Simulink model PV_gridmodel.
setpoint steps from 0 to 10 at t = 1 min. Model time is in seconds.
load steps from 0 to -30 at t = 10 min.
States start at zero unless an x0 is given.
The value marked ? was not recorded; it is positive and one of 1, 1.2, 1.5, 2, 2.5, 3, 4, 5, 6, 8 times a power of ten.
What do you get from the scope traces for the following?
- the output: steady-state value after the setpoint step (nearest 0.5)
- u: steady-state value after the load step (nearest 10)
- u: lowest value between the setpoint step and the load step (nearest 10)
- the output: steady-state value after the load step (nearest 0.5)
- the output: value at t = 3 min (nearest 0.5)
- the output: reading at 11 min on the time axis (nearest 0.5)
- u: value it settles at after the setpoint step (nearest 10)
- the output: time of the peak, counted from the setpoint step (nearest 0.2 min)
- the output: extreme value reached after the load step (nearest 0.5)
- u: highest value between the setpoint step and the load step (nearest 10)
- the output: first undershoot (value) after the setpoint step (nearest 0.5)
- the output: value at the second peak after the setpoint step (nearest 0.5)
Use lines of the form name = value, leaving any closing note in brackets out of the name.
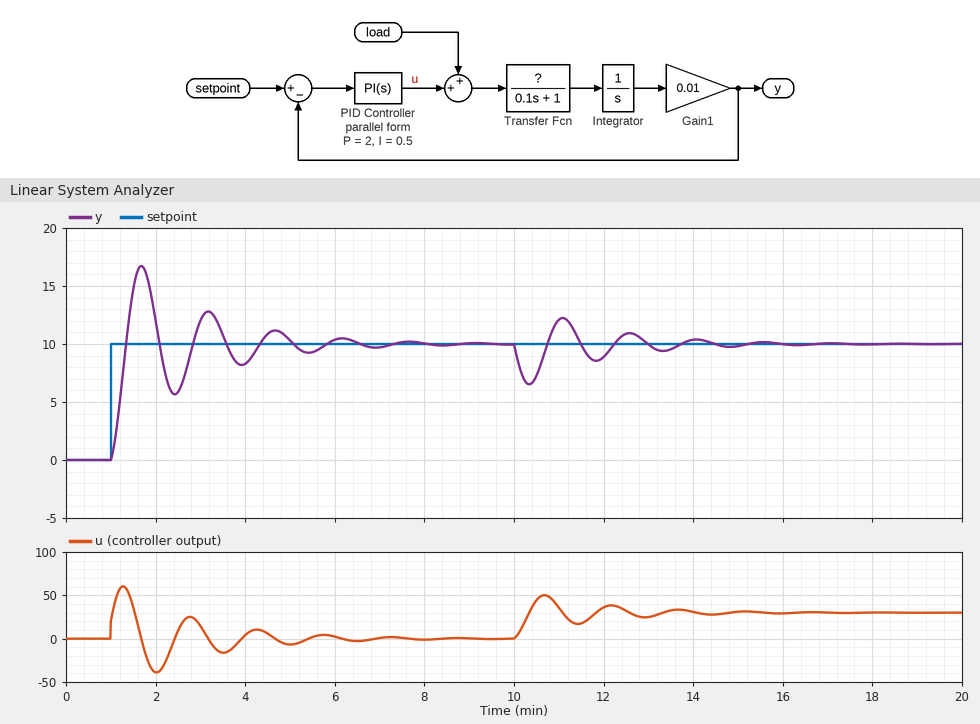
the output: steady-state value after the setpoint step = 10.0
u: steady-state value after the load step = 30
u: lowest value between the setpoint step and the load step = -40
the output: steady-state value after the load step = 10.0
the output: value at t = 3 min = 12.0
the output: reading at 11 min on the time axis = 12.0
u: value it settles at after the setpoint step = 0
the output: time of the peak, counted from the setpoint step = 0.6 min
the output: extreme value reached after the load step = 6.5
u: highest value between the setpoint step and the load step = 60
the output: first undershoot (value) after the setpoint step = 5.5
the output: value at the second peak after the setpoint step = 13.0
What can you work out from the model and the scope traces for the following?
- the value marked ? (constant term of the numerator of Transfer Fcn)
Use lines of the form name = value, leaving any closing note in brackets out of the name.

the value marked ? = 1
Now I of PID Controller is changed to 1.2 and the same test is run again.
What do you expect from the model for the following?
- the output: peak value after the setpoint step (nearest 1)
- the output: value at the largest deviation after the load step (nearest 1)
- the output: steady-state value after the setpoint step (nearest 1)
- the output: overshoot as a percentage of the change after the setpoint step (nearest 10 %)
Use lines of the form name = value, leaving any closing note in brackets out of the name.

the output: peak value after the setpoint step = 18
the output: value at the largest deviation after the load step = 8
the output: steady-state value after the setpoint step = 10
the output: overshoot as a percentage of the change after the setpoint step = 80 %
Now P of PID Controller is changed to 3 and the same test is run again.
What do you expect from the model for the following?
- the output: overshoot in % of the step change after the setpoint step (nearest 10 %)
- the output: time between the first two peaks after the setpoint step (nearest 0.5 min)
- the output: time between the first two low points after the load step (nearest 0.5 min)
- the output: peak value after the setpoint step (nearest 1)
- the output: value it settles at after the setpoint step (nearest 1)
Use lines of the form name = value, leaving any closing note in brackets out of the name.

the output: overshoot in % of the step change after the setpoint step = 60 %
the output: time between the first two peaks after the setpoint step = 1.5 min
the output: time between the first two low points after the load step = 1.5 min
the output: peak value after the setpoint step = 16
the output: value it settles at after the setpoint step = 10
